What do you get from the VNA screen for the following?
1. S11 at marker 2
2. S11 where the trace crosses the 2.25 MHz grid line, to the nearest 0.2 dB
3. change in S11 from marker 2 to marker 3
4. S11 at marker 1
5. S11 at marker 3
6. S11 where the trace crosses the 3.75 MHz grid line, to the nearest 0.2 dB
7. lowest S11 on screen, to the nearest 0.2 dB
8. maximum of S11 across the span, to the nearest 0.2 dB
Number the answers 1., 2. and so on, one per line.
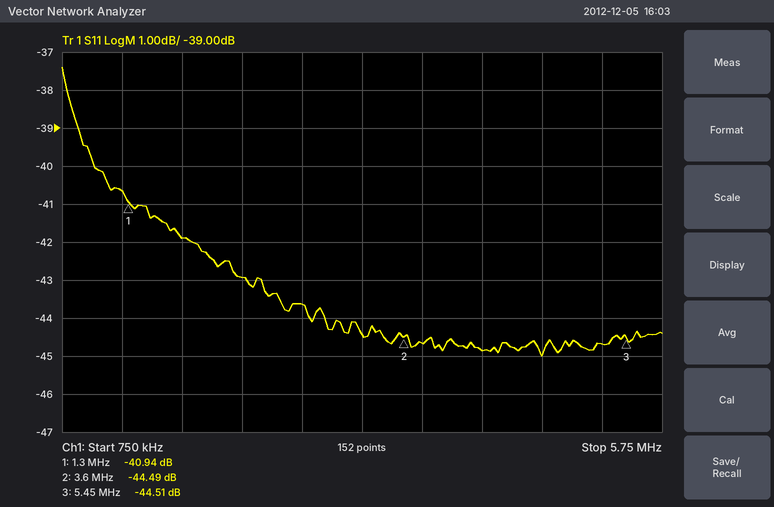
1. -44.49 dB
2. -43.0 dB
3. -0.02 dB
4. -40.94 dB
5. -44.51 dB
6. -44.6 dB
7. -45.0 dB
8. -37.4 dB
